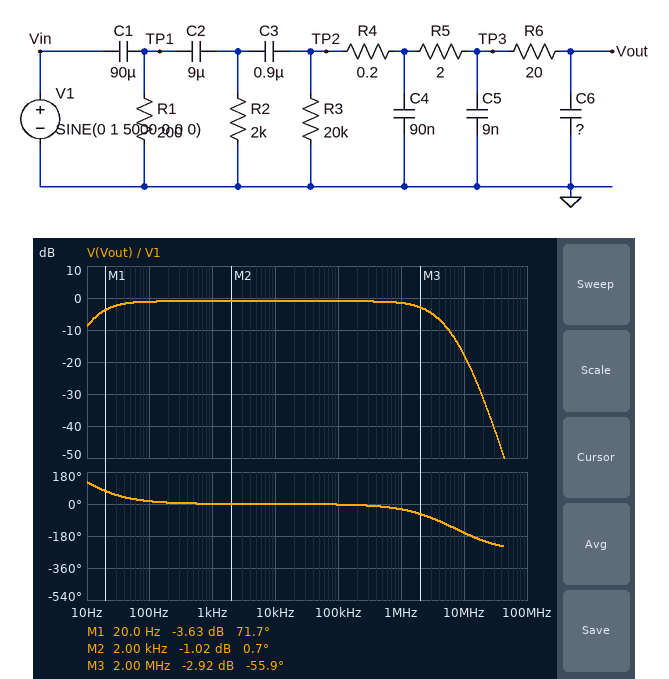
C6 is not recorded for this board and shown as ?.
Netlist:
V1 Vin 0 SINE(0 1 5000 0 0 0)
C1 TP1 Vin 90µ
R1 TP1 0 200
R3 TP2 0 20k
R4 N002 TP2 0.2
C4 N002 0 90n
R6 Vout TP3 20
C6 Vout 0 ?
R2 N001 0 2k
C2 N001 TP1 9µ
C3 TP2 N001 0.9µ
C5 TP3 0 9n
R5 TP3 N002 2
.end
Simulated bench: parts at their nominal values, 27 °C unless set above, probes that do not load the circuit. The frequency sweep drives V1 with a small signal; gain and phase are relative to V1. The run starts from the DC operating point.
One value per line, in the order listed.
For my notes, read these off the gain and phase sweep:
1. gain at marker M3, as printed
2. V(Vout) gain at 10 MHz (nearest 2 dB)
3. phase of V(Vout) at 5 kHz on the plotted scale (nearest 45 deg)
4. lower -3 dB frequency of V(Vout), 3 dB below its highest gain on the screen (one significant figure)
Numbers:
-2.92 dB
-18 dB
0 deg
20 Hz
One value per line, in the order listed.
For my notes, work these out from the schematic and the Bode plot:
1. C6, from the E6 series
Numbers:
2.2 nF
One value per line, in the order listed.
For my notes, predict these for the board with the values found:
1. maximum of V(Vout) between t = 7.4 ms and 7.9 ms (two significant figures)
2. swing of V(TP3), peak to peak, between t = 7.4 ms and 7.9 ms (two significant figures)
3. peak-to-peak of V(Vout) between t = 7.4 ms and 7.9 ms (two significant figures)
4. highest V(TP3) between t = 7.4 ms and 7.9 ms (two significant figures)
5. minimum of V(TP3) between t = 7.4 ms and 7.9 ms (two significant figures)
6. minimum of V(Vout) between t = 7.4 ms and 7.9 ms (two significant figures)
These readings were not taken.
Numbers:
890 mV
1.8 V
1.8 V
890 mV
-890 mV
-890 mV
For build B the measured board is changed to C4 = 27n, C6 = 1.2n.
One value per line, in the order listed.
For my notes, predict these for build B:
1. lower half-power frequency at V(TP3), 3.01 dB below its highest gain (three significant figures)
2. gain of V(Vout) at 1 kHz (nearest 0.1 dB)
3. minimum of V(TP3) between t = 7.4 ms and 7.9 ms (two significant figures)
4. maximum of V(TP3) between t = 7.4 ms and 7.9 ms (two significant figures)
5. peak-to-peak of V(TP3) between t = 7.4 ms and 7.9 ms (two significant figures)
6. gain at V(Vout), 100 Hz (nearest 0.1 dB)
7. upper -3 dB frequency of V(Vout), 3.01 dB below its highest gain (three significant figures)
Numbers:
18.9 Hz
-0.4 dB
-960 mV
950 mV
1.9 V
-0.5 dB
4.23 MHz
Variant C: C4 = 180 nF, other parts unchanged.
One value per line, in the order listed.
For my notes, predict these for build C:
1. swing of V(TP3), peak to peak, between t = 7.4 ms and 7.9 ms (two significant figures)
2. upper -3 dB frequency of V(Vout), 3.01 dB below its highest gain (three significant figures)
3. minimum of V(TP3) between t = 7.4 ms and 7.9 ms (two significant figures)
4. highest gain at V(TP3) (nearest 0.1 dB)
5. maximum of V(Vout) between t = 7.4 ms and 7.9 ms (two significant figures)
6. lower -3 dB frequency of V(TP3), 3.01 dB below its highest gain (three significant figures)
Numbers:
1.6 V
2.35 MHz
-810 mV
-1.8 dB
810 mV
17.8 Hz
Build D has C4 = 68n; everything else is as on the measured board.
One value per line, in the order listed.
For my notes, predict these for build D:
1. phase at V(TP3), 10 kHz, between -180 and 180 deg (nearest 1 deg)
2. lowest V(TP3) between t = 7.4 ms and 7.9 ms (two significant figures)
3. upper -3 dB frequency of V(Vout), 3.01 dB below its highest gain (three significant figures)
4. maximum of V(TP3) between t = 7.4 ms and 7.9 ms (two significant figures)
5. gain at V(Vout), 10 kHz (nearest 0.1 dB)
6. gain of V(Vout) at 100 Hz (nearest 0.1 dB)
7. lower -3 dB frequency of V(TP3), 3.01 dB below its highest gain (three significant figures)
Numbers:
0 deg
-910 mV
2.70 MHz
910 mV
-0.8 dB
-0.9 dB
18.6 Hz
